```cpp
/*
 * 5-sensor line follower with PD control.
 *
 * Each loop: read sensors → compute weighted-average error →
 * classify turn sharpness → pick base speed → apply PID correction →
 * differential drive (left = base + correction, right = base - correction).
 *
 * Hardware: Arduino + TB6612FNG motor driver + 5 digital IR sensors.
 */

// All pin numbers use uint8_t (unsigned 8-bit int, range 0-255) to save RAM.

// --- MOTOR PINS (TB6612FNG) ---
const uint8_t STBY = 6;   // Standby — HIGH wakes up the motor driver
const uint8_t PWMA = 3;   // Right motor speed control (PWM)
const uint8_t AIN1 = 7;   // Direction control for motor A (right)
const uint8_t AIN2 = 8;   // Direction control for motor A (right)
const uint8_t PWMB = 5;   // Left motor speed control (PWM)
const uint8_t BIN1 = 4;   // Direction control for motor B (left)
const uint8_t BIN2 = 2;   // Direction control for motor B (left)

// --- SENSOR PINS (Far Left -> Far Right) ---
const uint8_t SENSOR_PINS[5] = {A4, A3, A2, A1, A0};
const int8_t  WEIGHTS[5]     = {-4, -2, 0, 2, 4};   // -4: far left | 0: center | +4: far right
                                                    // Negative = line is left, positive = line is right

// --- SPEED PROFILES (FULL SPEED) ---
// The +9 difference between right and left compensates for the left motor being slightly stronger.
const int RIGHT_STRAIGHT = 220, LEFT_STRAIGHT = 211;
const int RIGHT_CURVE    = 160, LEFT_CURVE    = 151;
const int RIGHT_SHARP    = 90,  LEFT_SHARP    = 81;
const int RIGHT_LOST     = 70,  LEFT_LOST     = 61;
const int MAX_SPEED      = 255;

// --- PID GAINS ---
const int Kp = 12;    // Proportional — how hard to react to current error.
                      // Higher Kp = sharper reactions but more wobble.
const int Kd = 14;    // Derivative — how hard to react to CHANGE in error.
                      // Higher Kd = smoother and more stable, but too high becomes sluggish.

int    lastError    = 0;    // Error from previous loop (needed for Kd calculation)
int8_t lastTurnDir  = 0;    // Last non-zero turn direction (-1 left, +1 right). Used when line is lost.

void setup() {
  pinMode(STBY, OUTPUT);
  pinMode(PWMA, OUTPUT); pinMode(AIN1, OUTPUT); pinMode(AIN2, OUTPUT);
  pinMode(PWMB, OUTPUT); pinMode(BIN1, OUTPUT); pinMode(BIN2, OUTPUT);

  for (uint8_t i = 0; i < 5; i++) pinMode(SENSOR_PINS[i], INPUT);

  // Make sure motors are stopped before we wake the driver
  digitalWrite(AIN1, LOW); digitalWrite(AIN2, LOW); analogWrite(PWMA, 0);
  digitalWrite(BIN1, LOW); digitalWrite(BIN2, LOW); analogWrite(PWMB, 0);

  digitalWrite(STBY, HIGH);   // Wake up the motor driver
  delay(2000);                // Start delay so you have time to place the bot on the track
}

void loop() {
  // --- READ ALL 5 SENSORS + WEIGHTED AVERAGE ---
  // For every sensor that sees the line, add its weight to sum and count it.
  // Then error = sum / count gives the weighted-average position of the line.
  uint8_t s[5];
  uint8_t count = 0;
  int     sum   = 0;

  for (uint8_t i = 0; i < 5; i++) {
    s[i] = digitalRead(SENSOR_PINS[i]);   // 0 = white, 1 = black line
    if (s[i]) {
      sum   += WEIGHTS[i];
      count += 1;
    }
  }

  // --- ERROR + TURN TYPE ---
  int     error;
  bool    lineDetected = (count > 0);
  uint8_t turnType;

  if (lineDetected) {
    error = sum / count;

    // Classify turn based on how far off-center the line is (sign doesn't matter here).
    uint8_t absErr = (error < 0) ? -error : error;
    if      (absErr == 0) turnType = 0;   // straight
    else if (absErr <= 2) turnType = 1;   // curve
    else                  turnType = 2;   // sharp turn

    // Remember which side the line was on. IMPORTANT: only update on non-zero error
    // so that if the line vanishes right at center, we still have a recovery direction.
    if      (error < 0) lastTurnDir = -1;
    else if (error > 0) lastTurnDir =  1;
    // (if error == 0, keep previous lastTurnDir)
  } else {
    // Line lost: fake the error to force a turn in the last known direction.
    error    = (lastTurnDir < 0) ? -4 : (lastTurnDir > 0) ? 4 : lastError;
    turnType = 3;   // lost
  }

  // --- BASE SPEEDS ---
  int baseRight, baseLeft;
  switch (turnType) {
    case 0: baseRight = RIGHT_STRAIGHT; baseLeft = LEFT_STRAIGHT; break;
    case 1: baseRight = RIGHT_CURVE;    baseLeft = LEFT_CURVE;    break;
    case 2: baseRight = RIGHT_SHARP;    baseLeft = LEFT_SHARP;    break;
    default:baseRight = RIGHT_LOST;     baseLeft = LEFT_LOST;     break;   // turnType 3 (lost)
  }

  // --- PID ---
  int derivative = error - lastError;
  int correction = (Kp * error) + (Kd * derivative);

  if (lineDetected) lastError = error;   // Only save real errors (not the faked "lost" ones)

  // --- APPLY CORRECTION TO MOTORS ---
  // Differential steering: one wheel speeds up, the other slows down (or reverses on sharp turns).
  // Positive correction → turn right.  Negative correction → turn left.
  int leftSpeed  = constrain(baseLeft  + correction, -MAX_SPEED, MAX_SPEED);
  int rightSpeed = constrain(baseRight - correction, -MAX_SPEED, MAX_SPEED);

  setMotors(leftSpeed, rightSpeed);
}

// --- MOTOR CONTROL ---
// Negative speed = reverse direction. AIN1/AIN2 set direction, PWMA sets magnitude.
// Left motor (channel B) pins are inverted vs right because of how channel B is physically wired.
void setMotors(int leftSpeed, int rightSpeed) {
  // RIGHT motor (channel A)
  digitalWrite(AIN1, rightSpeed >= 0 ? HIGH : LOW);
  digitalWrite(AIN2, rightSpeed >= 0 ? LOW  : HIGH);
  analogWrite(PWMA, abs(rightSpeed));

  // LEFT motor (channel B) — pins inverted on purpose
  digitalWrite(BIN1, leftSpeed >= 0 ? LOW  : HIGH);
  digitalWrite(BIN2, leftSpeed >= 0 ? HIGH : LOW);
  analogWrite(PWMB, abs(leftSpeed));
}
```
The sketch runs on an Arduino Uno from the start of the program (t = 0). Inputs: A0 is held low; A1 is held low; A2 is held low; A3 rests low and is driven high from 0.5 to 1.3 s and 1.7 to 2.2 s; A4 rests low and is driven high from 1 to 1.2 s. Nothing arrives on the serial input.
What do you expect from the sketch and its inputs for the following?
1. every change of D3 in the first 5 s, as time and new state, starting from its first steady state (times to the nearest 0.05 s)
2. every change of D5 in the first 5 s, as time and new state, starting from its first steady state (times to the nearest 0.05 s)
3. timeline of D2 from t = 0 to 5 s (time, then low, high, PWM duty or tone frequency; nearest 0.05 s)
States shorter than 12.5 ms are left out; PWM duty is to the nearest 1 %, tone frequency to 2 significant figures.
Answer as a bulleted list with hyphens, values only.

- 0 s low; 2 s PWM 72 %; 2.2 s PWM 57 %
- 0 s low; 2 s PWM 50 %; 2.2 s PWM 6 %
- 0 s low; 2 s high; 2.2 s low
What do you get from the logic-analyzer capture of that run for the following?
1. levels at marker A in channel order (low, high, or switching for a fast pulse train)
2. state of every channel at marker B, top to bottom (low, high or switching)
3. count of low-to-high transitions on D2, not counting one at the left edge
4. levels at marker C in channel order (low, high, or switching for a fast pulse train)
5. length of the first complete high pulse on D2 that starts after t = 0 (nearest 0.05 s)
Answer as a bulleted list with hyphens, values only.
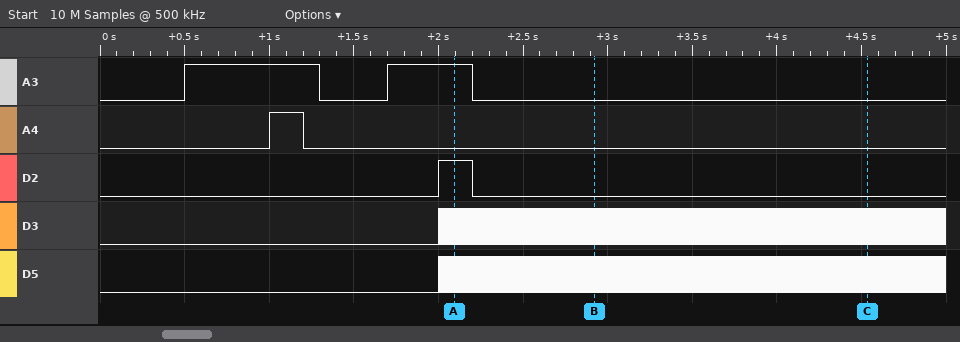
- A3 high, A4 low, D2 high, D3 switching, D5 switching
- A3 low, A4 low, D2 low, D3 switching, D5 switching
- 1
- A3 low, A4 low, D2 low, D3 switching, D5 switching
- 0.20 s
